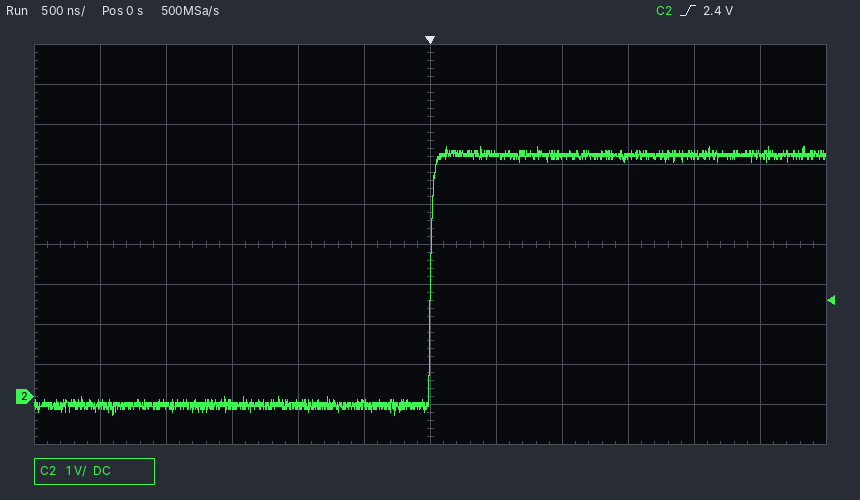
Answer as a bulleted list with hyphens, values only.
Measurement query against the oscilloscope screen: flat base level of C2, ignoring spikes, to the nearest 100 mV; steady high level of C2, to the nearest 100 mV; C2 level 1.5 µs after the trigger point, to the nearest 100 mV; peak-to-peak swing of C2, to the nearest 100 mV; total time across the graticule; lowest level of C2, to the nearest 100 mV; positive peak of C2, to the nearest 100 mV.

- -200 mV
- 6.0 V
- 6.0 V
- 6.7 V
- 6 µs
- -500 mV
- 6.2 V
